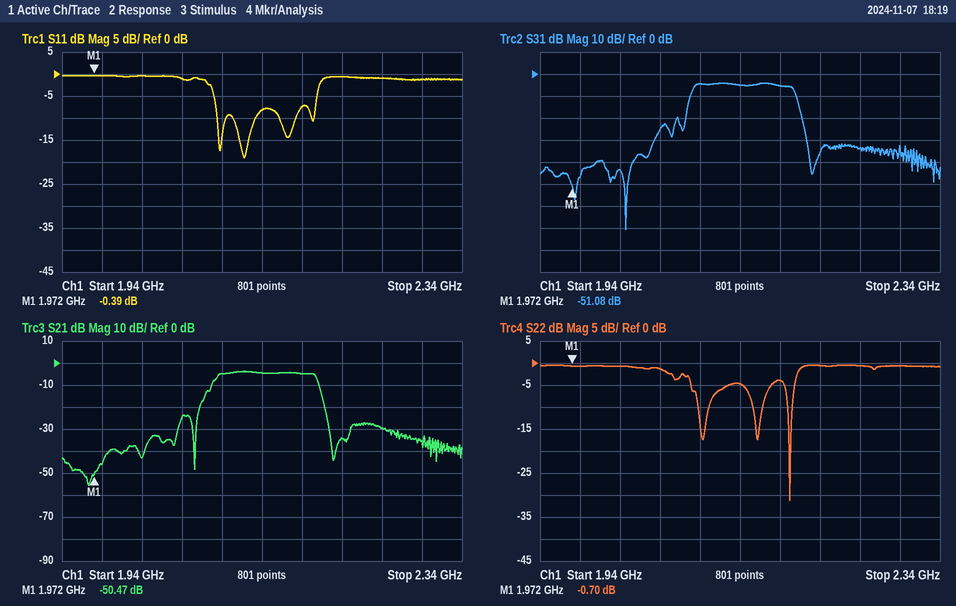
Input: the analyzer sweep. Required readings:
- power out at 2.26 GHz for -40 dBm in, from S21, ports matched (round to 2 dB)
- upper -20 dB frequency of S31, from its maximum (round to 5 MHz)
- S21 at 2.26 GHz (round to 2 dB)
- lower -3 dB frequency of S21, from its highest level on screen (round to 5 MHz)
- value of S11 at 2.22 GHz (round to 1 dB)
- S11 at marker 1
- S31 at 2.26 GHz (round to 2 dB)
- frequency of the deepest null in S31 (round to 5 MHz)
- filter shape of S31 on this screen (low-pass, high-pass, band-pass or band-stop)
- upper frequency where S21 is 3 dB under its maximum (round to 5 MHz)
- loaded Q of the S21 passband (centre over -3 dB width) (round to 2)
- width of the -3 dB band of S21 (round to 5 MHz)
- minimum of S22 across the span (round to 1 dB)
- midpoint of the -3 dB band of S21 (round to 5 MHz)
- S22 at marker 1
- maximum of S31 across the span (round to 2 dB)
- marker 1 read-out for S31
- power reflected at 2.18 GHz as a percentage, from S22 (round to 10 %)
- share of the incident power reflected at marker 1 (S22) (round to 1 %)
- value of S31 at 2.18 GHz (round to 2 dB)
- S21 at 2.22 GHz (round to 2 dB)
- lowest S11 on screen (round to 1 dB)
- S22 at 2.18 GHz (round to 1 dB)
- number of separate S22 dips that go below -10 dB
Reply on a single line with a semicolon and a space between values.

-70 dBm; 2.205 GHz; -30 dB; 2.095 GHz; -1 dB; -0.39 dB; -34 dB; 2.025 GHz; band-pass; 2.195 GHz; 22; 100 MHz; -31 dB; 2.145 GHz; -0.70 dB; -4 dB; -51.08 dB; 40 %; 85 %; -6 dB; -34 dB; -19 dB; -4 dB; 3
